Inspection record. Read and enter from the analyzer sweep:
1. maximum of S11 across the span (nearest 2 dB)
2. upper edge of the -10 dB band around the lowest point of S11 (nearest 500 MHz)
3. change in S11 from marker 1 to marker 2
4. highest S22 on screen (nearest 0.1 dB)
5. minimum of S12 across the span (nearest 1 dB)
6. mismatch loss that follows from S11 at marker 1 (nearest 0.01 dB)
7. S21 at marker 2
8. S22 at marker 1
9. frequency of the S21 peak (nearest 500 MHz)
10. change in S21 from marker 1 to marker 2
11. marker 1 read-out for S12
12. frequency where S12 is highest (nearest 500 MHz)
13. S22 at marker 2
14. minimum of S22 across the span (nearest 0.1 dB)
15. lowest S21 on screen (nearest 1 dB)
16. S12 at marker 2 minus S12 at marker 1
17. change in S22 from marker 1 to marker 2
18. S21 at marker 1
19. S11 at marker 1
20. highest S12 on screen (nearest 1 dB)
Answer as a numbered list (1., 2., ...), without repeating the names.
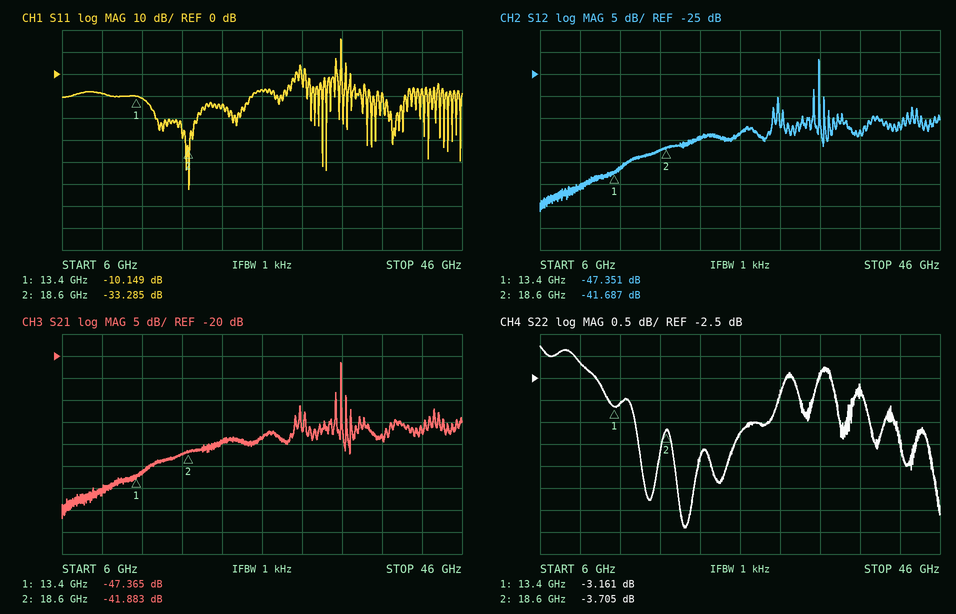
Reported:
1. 16 dB
2. 25.0 GHz
3. -23.136 dB
4. -1.8 dB
5. -56 dB
6. 0.44 dB
7. -41.883 dB
8. -3.161 dB
9. 34.0 GHz
10. 5.482 dB
11. -47.351 dB
12. 34.0 GHz
13. -3.705 dB
14. -5.9 dB
15. -57 dB
16. 5.664 dB
17. -0.544 dB
18. -47.365 dB
19. -10.149 dB
20. -22 dB
